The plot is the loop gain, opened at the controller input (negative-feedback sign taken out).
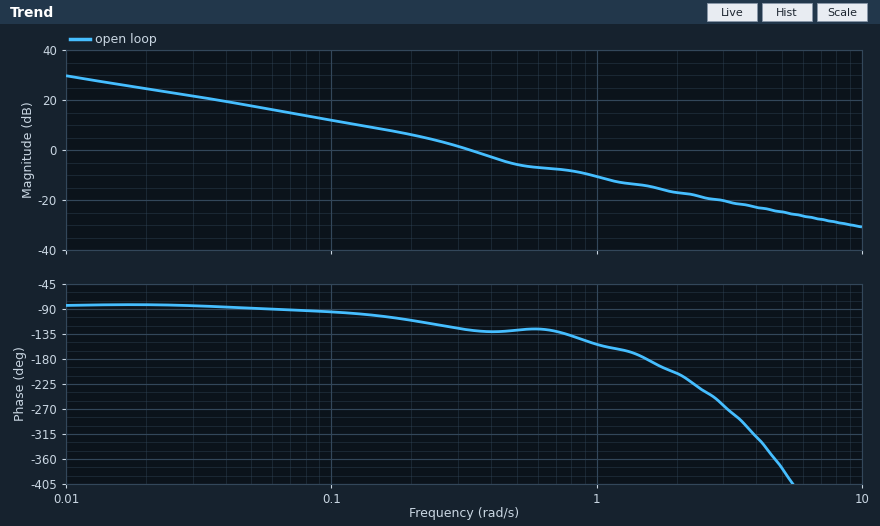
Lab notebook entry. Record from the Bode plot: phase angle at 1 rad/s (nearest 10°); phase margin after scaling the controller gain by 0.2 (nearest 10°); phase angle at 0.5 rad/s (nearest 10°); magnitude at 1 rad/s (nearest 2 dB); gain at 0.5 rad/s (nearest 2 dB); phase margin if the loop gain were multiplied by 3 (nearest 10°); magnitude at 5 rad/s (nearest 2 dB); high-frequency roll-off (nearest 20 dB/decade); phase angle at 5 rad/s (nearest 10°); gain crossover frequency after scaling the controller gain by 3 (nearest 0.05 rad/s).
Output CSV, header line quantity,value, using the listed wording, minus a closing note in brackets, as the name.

quantity,value
phase angle at 1 rad/s,-150°
phase margin after scaling the controller gain by 0.2,90°
phase angle at 0.5 rad/s,-130°
magnitude at 1 rad/s,-10 dB
gain at 0.5 rad/s,-6 dB
phase margin if the loop gain were multiplied by 3,30°
magnitude at 5 rad/s,-24 dB
high-frequency roll-off,-20 dB/decade
phase angle at 5 rad/s,-380°
gain crossover frequency after scaling the controller gain by 3,0.90 rad/s
